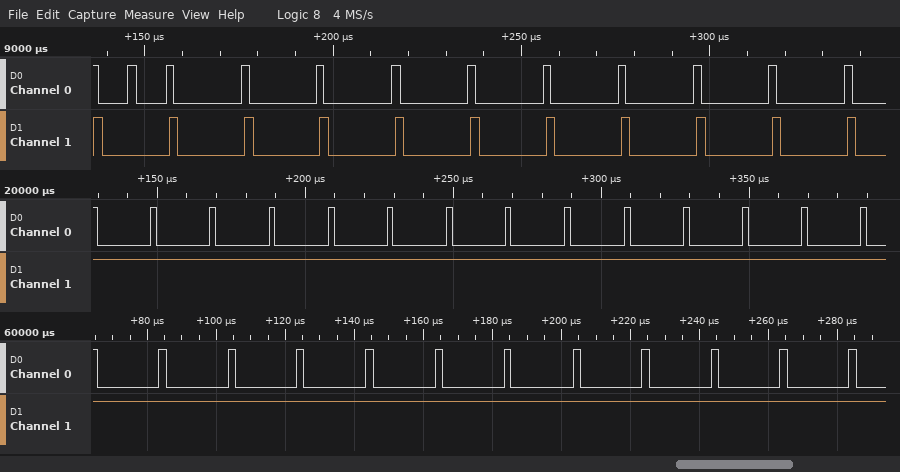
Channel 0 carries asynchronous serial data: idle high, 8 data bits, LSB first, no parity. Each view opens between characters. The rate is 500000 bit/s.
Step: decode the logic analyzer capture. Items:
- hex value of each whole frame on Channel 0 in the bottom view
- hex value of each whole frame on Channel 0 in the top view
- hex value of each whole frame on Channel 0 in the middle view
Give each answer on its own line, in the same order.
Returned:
00, 00, 00, 00, 00, 00, 00, 00, 00, 00, 00
08, 00, 00, 00, 00, 00, 00, 00, 00, 00
00, 00, 00, 00, 00, 00, 00, 00, 00, 00, 00, 00, 00
